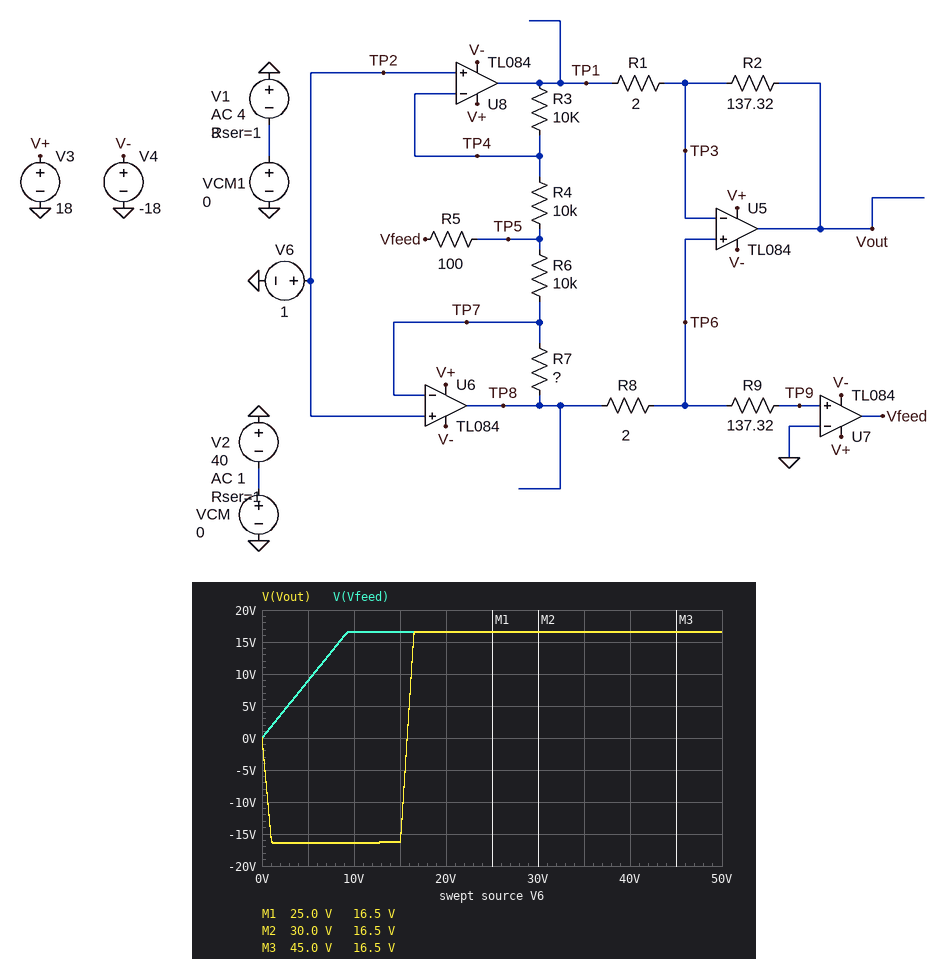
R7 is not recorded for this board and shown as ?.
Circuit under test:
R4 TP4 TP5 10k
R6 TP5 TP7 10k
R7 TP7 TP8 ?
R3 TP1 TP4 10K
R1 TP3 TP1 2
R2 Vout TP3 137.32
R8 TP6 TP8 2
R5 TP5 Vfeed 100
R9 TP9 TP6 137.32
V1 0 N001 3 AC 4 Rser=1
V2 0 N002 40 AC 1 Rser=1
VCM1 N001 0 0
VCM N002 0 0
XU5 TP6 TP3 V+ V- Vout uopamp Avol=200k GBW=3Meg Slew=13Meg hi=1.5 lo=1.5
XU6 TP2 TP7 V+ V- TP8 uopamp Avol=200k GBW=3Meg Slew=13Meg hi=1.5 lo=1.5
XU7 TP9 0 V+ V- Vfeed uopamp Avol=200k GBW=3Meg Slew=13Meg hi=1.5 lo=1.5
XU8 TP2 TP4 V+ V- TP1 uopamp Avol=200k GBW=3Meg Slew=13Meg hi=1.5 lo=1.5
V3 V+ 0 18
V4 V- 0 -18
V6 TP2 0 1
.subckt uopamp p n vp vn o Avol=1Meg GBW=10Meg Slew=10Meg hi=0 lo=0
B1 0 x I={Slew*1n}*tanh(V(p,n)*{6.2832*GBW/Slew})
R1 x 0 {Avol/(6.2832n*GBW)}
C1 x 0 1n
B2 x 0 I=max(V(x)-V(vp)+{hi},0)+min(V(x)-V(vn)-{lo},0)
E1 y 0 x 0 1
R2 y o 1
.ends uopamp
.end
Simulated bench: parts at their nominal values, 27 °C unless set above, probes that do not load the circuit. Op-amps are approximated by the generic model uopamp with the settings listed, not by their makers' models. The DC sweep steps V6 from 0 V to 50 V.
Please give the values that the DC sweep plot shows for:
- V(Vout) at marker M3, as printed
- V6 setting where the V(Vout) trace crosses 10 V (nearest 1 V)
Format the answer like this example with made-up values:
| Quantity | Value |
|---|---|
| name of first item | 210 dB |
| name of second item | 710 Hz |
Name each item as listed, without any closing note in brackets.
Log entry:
| Quantity | Value |
|---|---|
| V(Vout) at marker M3, as printed | 16.5 V |
| V6 setting where the V(Vout) trace crosses 10 V | 16 V |
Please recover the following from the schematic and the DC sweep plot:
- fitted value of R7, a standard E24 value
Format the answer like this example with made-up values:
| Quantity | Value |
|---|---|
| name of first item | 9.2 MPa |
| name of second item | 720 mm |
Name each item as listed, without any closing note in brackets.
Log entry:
| Quantity | Value |
|---|---|
| fitted value of R7, a standard E24 value | 13 kΩ |
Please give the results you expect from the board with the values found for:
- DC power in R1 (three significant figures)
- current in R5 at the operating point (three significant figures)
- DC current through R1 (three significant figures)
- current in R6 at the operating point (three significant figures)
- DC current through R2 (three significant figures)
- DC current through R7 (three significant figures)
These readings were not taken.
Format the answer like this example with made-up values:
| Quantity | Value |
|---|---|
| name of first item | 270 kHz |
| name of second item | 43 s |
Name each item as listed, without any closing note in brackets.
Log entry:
| Quantity | Value |
|---|---|
| DC power in R1 | 26.6 mW |
| current in R5 at the operating point | 154 µA |
| DC current through R1 | 115 mA |
| current in R6 at the operating point | 76.9 µA |
| DC current through R2 | 115 mA |
| DC current through R7 | 76.9 µA |
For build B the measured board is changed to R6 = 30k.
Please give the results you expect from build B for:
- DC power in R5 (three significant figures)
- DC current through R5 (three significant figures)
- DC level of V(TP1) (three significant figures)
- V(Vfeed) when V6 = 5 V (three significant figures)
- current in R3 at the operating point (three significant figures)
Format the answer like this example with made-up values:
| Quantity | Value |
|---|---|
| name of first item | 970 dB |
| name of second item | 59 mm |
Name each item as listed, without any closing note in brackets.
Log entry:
| Quantity | Value |
|---|---|
| DC power in R5 | 9.47 µW |
| DC current through R5 | 308 µA |
| DC level of V(TP1) | -1.31 V |
| V(Vfeed) when V6 = 5 V | 16.5 V |
| current in R3 at the operating point | 231 µA |
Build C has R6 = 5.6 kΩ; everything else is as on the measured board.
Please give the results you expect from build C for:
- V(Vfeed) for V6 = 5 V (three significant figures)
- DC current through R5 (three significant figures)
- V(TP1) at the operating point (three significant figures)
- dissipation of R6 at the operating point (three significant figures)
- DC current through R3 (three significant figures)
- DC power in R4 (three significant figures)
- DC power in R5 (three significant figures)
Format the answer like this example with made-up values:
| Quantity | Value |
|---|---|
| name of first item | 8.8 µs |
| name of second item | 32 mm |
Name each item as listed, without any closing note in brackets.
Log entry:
| Quantity | Value |
|---|---|
| V(Vfeed) for V6 = 5 V | 7.21 V |
| DC current through R5 | 120 µA |
| V(TP1) at the operating point | 569 mV |
| dissipation of R6 at the operating point | 33.1 µW |
| DC current through R3 | 43.1 µA |
| DC power in R4 | 18.6 µW |
| DC power in R5 | 1.44 µW |
